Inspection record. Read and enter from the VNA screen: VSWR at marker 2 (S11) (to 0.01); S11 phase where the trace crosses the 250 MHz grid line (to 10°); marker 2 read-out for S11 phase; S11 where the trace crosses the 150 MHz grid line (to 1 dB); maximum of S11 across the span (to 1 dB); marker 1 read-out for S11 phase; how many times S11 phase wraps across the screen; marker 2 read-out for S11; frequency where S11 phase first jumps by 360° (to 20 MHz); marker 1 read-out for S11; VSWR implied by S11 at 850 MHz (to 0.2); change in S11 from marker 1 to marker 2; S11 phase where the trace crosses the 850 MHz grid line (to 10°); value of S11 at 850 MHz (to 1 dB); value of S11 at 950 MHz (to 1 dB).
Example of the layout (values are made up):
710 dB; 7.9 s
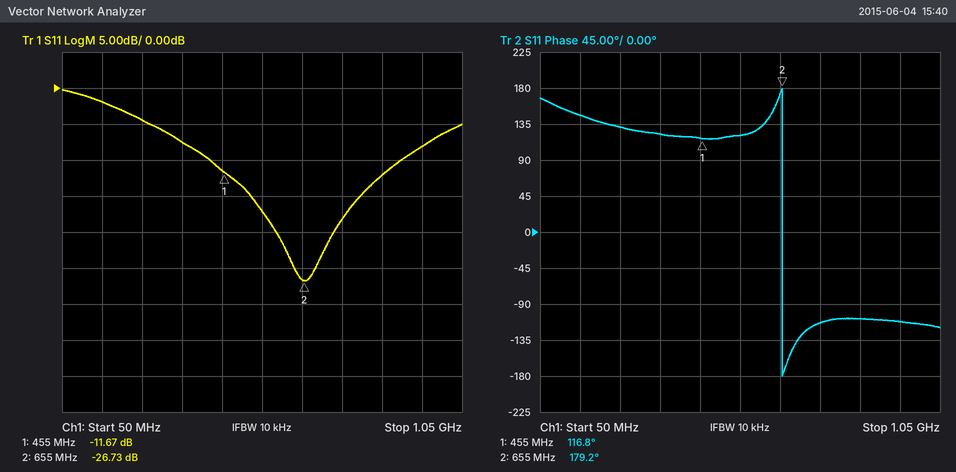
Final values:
1.10; 130°; 179.2°; -2 dB; 0 dB; 116.8°; 1; -26.73 dB; 660 MHz; -11.67 dB; 1.6; -15.06 dB; -110°; -12 dB; -8 dB
